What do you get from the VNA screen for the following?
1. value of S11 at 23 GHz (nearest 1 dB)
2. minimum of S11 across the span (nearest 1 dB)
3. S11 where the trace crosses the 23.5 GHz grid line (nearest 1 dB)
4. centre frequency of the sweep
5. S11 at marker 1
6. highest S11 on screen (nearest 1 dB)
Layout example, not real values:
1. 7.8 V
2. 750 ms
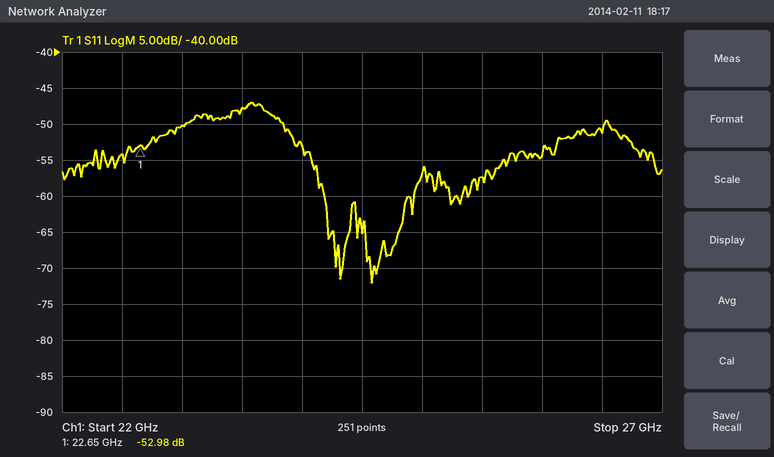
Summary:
1. -50 dB
2. -72 dB
3. -48 dB
4. 24.5 GHz
5. -52.98 dB
6. -47 dB
